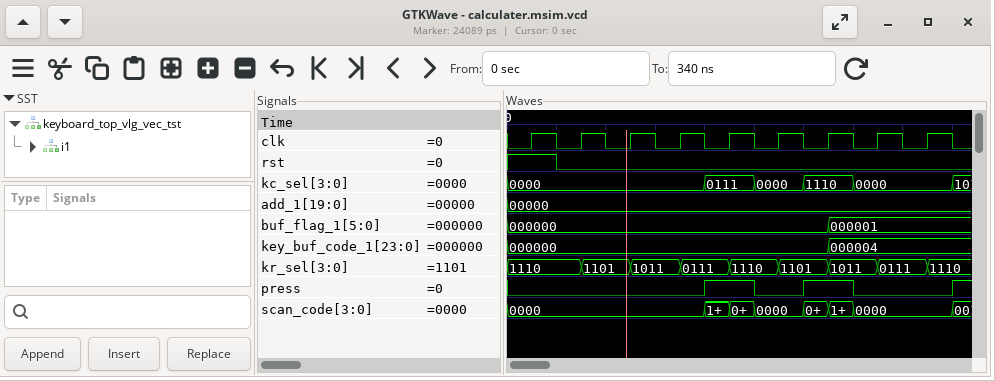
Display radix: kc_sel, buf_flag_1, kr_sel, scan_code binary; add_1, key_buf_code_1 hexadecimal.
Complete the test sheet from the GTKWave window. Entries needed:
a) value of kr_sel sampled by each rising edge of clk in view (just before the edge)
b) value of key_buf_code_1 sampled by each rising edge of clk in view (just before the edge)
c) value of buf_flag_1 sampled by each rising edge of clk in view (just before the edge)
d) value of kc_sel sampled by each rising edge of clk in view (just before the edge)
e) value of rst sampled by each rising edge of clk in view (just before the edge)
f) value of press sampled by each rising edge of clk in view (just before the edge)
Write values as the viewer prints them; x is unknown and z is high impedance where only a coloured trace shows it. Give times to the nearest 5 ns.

1110, 1110, 1101, 1011, 0111, 1110, 1101, 1011, 0111
000000, 000000, 000000, 000000, 000000, 000000, 000000, 000004, 000004
000000, 000000, 000000, 000000, 000000, 000000, 000000, 000001, 000001
0000, 0000, 0000, 0000, 0111, 0000, 1110, 0000, 0000
1 0 0 0 0 0 0 0 0
0 0 0 0 1 0 1 0 0
